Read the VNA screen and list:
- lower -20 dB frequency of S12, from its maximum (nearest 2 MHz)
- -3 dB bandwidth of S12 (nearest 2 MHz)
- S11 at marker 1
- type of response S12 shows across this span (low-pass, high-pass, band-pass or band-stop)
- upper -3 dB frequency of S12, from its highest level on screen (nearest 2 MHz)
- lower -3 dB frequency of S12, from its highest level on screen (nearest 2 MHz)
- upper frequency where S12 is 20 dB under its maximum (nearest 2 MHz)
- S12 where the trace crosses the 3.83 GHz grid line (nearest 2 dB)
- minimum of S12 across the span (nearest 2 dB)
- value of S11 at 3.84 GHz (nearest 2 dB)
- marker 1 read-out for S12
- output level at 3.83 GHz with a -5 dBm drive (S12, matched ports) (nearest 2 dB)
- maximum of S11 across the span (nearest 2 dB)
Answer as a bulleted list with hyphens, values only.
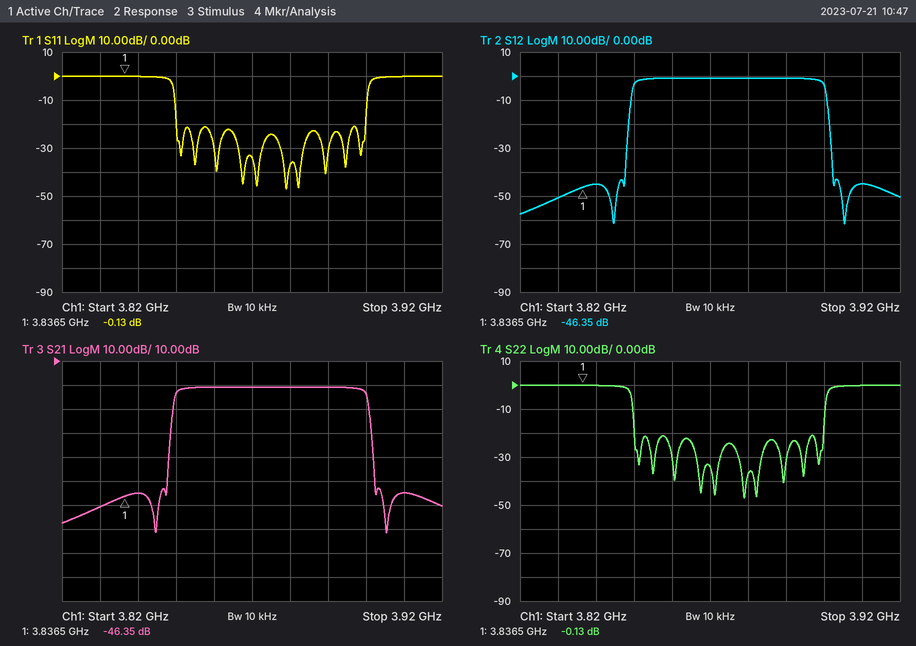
- 3.848 GHz
- 50 MHz
- -0.13 dB
- band-pass
- 3.900 GHz
- 3.850 GHz
- 3.902 GHz
- -50 dB
- -62 dB
- 0 dB
- -46.35 dB
- -56 dBm
- 0 dB
